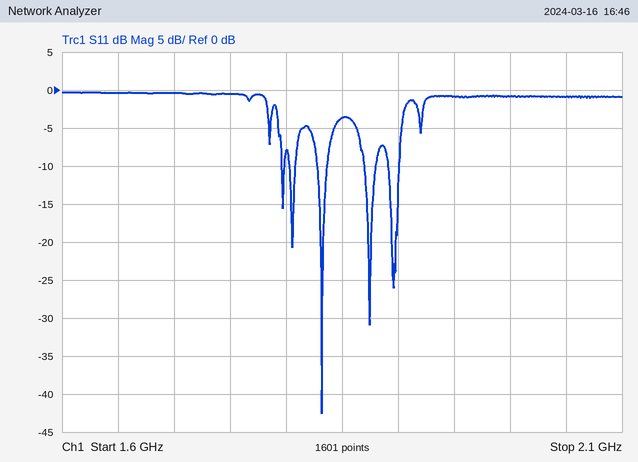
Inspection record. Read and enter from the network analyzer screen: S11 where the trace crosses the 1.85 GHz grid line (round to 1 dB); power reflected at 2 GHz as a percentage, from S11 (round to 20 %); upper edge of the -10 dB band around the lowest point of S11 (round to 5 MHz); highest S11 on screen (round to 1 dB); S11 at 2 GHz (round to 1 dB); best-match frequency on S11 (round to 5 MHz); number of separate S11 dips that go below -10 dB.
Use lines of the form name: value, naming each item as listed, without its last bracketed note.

S11 where the trace crosses the 1.85 GHz grid line: -4 dB
power reflected at 2 GHz as a percentage, from S11: 80 %
upper edge of the -10 dB band around the lowest point of S11: 1.835 GHz
highest S11 on screen: 0 dB
S11 at 2 GHz: -1 dB
best-match frequency on S11: 1.830 GHz
number of separate S11 dips that go below -10 dB: 5
